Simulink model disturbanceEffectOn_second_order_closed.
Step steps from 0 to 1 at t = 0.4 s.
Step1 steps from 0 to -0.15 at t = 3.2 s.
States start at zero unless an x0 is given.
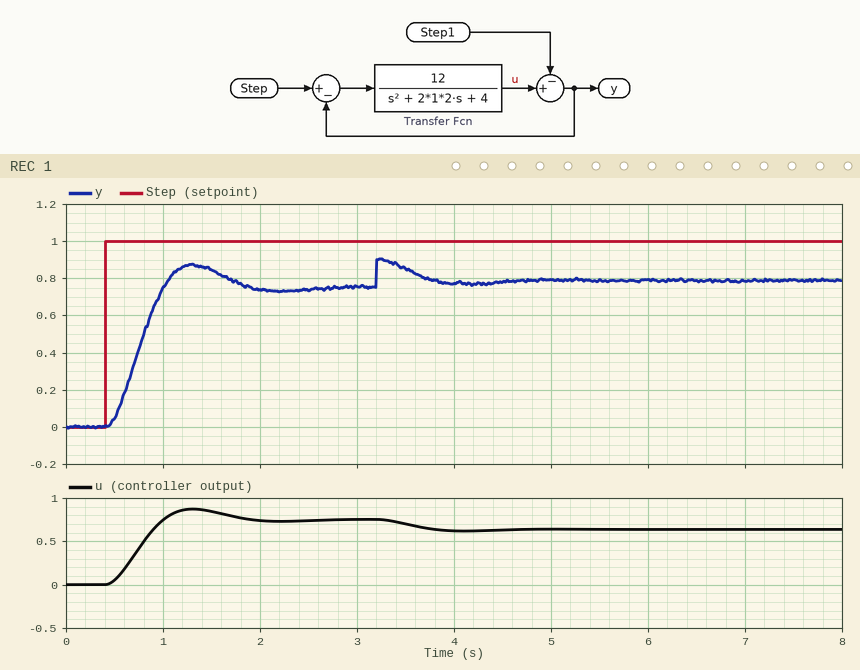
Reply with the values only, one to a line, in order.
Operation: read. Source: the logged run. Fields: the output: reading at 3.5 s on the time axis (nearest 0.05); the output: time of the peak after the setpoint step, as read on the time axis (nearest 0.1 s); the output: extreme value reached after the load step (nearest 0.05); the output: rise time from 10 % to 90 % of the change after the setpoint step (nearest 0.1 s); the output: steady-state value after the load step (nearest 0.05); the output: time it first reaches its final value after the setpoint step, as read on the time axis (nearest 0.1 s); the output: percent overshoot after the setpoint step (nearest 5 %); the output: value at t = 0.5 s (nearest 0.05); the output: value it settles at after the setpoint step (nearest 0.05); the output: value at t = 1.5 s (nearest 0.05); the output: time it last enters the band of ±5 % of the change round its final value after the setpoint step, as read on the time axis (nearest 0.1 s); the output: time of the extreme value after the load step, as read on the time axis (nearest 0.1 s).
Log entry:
0.85
1.3 s
0.90
0.4 s
0.80
1.0 s
15 %
0.05
0.75
0.85
1.7 s
3.2 s
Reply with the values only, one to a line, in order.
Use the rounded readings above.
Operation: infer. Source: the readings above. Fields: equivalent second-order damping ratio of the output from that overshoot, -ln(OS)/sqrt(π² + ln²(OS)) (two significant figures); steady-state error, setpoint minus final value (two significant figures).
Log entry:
0.52
0.25
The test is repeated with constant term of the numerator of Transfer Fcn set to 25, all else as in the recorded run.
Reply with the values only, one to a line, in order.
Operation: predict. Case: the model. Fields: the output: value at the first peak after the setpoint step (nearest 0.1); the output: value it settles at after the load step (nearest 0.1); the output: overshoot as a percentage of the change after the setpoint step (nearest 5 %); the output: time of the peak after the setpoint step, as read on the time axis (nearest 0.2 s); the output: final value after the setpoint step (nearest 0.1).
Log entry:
1.1
0.9
30 %
1.0 s
0.9
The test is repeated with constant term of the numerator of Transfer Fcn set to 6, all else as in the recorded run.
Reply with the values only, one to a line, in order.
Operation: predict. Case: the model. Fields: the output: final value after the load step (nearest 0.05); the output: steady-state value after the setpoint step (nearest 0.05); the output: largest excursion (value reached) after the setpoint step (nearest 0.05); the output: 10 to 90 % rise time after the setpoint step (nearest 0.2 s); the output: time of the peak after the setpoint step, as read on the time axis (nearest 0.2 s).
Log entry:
0.65
0.60
0.65
0.6 s
1.6 s
